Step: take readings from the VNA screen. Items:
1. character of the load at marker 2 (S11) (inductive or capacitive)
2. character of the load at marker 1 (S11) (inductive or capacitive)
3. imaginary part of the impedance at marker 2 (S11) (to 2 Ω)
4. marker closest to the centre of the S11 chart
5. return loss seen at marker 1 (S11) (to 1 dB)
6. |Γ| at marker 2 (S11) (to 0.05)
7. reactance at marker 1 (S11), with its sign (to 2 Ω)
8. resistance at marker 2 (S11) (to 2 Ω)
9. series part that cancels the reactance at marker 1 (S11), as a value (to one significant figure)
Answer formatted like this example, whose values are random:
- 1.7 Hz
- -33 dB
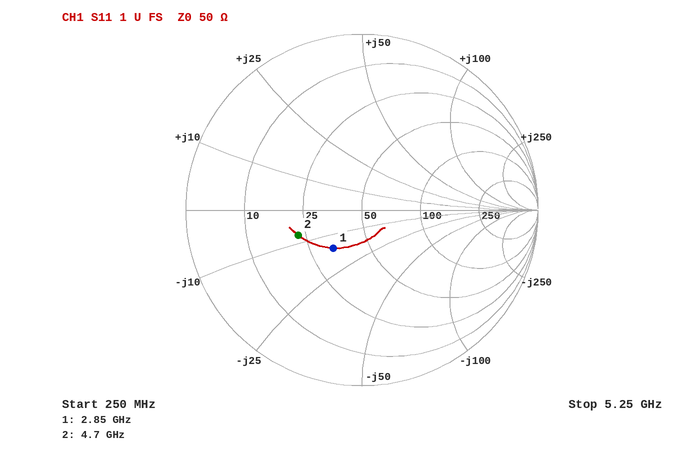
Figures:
- capacitive
- capacitive
- -8 Ω
- marker 1
- 11 dB
- 0.40
- -16 Ω
- 22 Ω
- 900 pH
